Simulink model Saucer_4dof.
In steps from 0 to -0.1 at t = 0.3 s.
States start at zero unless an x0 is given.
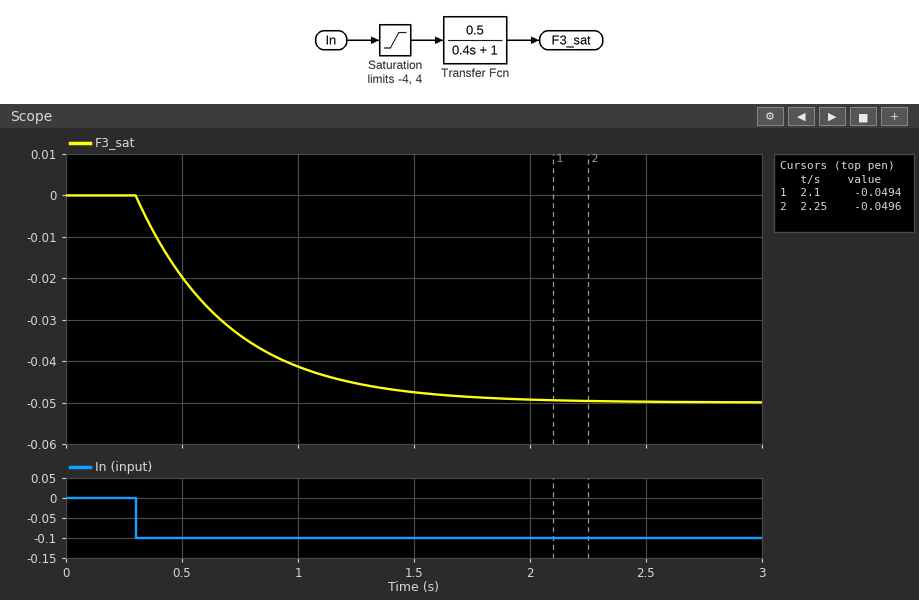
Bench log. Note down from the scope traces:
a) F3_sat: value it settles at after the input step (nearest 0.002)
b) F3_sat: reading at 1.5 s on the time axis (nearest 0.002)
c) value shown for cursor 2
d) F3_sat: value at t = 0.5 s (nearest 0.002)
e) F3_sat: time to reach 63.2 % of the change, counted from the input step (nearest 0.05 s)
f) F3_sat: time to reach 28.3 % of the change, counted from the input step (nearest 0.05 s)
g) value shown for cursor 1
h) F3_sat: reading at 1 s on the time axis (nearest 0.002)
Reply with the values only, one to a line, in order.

-0.050
-0.048
-0.0496
-0.020
0.40 s
0.15 s
-0.0494
-0.042
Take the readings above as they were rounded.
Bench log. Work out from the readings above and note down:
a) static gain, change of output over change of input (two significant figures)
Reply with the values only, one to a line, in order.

0.50
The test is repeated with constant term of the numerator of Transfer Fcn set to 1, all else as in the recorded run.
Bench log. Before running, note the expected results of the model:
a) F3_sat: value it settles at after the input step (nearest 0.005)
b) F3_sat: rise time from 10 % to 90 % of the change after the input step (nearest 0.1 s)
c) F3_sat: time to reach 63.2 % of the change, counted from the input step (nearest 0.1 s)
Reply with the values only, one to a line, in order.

-0.100
0.9 s
0.4 s
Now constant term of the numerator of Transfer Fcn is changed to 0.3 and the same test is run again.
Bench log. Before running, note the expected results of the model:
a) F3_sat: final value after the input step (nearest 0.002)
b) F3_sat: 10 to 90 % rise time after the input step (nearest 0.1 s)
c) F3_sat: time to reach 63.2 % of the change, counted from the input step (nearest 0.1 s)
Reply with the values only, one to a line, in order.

-0.030
0.9 s
0.4 s
